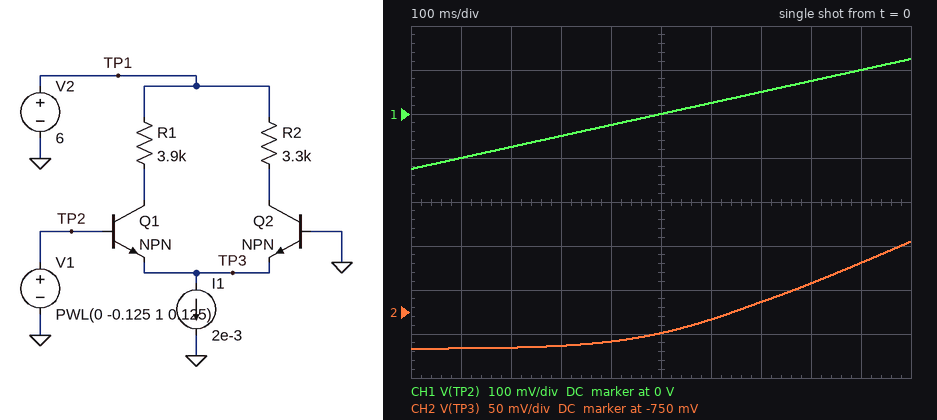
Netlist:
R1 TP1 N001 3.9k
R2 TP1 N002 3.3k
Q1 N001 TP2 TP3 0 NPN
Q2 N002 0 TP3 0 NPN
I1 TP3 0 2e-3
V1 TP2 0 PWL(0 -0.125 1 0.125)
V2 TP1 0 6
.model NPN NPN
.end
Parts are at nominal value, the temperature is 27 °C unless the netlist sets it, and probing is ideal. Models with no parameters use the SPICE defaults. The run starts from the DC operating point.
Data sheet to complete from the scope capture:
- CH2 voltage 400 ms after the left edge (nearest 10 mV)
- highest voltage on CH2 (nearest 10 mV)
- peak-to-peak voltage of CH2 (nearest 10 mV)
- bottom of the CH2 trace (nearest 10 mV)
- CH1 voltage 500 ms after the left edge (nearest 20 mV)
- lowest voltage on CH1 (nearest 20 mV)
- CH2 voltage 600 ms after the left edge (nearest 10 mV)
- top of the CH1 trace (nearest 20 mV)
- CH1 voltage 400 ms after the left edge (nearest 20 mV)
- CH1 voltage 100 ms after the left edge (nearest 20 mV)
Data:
-780 mV
-670 mV
120 mV
-790 mV
0 V
-120 mV
-760 mV
120 mV
-20 mV
-100 mV
